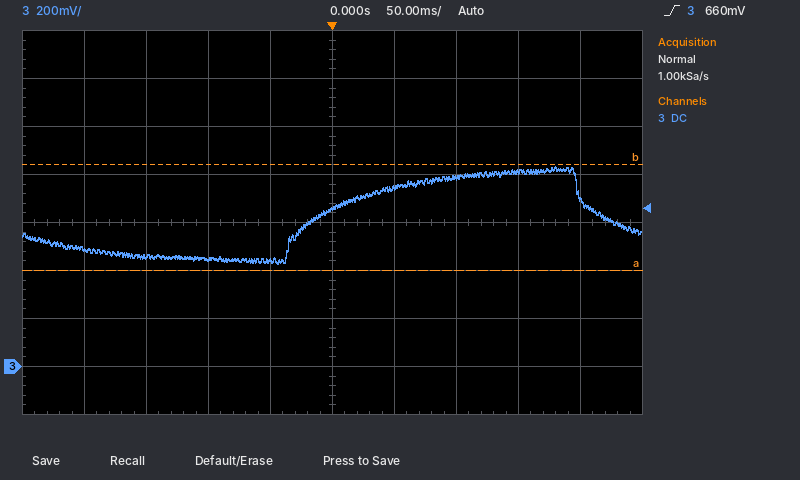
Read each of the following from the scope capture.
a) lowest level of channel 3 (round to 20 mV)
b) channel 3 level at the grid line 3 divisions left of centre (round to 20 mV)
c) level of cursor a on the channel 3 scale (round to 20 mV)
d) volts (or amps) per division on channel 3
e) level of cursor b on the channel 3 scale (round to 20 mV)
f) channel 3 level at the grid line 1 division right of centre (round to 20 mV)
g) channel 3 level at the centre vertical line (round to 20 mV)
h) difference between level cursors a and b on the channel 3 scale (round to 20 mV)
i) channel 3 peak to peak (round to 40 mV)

420 mV
460 mV
400 mV
200 mV
840 mV
740 mV
660 mV
440 mV
400 mV
